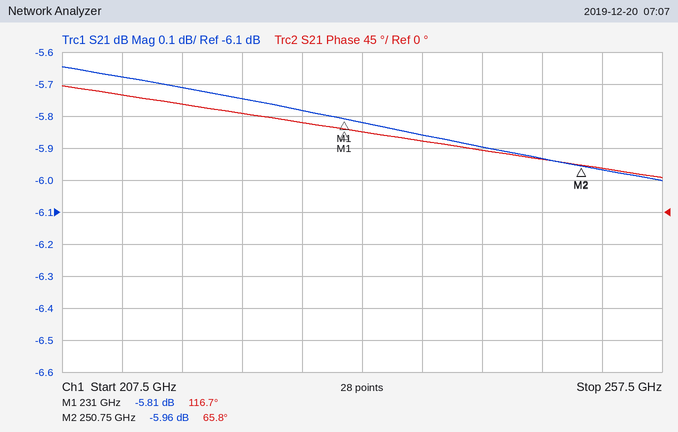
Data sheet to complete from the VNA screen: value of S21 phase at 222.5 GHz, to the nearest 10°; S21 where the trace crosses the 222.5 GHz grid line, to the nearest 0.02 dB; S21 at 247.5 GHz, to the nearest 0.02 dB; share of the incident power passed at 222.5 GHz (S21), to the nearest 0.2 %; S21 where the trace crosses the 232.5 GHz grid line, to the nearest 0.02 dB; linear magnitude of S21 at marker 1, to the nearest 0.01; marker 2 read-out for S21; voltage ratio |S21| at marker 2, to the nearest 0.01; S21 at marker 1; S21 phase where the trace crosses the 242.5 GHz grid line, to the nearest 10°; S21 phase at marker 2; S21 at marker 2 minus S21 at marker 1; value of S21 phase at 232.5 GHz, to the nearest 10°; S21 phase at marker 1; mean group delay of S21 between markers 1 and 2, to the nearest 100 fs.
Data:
140°
-5.74 dB
-5.94 dB
26.6 %
-5.82 dB
0.51
-5.96 dB
0.50
-5.81 dB
90°
65.8°
-0.15 dB
110°
116.7°
7.2 ps
